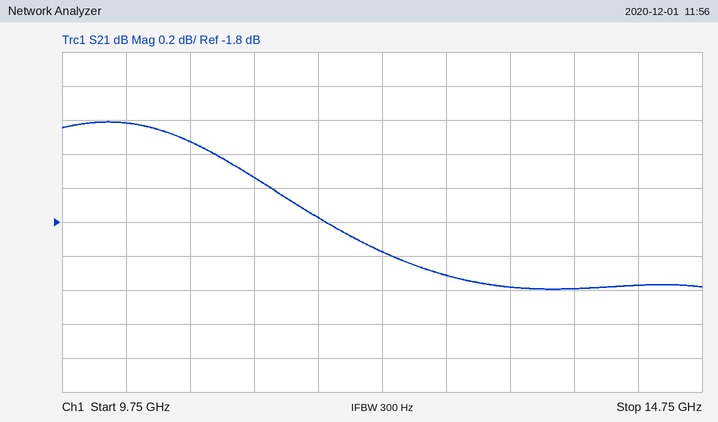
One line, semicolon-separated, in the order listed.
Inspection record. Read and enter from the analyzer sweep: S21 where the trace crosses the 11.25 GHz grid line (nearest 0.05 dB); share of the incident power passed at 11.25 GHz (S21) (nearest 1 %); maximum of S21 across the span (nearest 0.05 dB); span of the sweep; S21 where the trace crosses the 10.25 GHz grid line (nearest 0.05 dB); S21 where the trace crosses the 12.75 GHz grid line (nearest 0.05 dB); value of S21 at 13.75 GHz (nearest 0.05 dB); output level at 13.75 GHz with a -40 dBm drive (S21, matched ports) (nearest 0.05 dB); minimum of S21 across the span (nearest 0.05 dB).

-1.55 dB; 70 %; -1.20 dB; 5 GHz; -1.20 dB; -2.10 dB; -2.20 dB; -42.20 dBm; -2.20 dB
